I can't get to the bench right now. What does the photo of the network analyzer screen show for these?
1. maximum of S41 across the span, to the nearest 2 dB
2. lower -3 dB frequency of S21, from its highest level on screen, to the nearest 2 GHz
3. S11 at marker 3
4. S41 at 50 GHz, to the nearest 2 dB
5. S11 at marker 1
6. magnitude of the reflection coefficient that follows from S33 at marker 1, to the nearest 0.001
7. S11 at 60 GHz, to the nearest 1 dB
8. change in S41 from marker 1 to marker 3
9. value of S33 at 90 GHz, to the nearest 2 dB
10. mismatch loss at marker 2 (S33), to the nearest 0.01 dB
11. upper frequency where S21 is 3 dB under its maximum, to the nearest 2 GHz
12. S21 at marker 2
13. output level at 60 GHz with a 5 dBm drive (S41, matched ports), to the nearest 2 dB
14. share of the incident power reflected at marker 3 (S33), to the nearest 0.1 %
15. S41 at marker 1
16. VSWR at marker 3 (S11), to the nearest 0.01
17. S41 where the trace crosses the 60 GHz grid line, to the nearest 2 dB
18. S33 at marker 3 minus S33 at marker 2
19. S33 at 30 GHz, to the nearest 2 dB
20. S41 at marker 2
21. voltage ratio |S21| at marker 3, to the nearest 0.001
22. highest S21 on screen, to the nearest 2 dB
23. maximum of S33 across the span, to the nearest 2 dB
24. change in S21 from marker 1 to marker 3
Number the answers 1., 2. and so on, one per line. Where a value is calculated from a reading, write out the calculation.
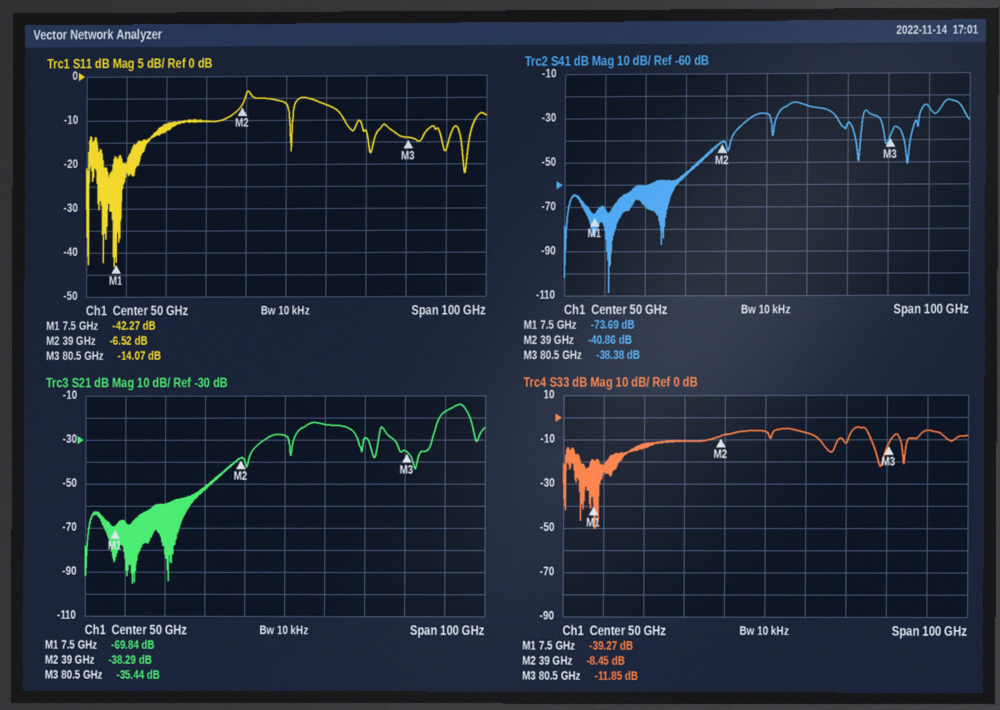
1. -22 dB
2. 90 GHz
3. -14.07 dB
4. -28 dB
5. -42.27 dB
6. 10^(-39.27/20) ≈ 0.011
7. -7 dB
8. -38.38 − (-73.69) = 35.31 dB
9. -6 dB
10. −10 log10(1 − 10^(-8.45/10)) ≈ 0.67 dB
11. 96 GHz
12. -38.29 dB
13. 5 dBm + (-24 dB) = -20 dBm
14. 10^(-11.85/10) ≈ 6.5 %
15. -73.69 dB
16. (1 + 0.1979)/(1 − 0.1979) ≈ 1.49
17. -24 dB
18. -11.85 − (-8.45) = -3.40 dB
19. -10 dB
20. -40.86 dB
21. 10^(-35.44/20) ≈ 0.017
22. -14 dB
23. -4 dB
24. -35.44 − (-69.84) = 34.40 dB
